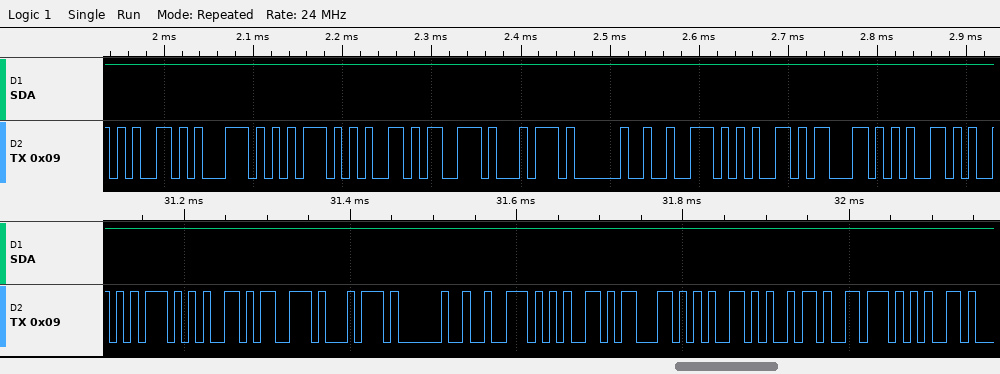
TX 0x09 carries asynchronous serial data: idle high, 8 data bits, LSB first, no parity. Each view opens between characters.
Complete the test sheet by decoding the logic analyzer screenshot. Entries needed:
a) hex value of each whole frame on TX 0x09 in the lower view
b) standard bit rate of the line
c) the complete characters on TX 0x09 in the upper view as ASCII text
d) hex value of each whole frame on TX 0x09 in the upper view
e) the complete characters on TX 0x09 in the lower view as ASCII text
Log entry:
75, 65, 73, 74, 20, 72, 65, 63, 65, 69, 76, 65
115200 baud
"equest rece"
65, 71, 75, 65, 73, 74, 20, 72, 65, 63, 65
"uest receive"
